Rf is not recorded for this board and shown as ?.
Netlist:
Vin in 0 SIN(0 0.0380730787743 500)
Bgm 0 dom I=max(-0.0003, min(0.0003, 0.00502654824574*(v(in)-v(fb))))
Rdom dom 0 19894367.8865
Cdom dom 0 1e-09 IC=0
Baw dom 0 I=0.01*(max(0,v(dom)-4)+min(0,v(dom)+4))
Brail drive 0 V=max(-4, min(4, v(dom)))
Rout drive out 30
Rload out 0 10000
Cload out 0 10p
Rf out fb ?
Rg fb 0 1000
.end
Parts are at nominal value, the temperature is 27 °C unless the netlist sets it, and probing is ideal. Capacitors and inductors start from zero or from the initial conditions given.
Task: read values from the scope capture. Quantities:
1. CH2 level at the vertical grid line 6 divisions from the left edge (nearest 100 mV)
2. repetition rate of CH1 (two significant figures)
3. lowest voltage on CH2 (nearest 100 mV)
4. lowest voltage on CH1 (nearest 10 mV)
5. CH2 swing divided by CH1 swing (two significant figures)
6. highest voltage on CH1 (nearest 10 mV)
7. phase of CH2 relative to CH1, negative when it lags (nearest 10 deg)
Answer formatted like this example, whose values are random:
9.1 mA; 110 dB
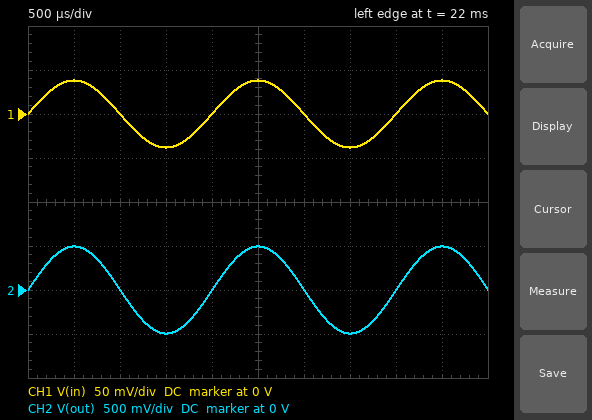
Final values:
0 V; 500 Hz; -500 mV; -40 mV; 13; 40 mV; 0 deg
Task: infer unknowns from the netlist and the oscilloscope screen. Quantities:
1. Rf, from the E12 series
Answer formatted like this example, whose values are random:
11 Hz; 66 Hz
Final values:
12 kΩ
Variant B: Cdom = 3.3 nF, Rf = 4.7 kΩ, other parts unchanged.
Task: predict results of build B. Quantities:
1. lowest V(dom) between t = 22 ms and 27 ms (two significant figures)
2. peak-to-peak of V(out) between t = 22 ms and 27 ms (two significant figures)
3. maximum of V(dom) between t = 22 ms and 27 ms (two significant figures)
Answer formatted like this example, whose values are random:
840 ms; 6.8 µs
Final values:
-220 mV; 430 mV; 220 mV
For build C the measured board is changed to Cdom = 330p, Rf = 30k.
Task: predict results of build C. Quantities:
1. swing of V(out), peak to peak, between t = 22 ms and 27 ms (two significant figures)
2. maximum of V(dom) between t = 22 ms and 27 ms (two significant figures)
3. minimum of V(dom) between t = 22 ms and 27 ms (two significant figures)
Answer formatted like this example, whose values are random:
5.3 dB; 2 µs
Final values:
2.4 V; 1.2 V; -1.2 V
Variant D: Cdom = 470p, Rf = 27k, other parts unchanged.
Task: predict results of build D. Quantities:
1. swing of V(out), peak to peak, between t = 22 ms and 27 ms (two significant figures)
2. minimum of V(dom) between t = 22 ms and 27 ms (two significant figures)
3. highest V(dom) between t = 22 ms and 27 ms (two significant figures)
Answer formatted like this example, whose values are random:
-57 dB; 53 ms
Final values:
2.1 V; -1.1 V; 1.1 V
